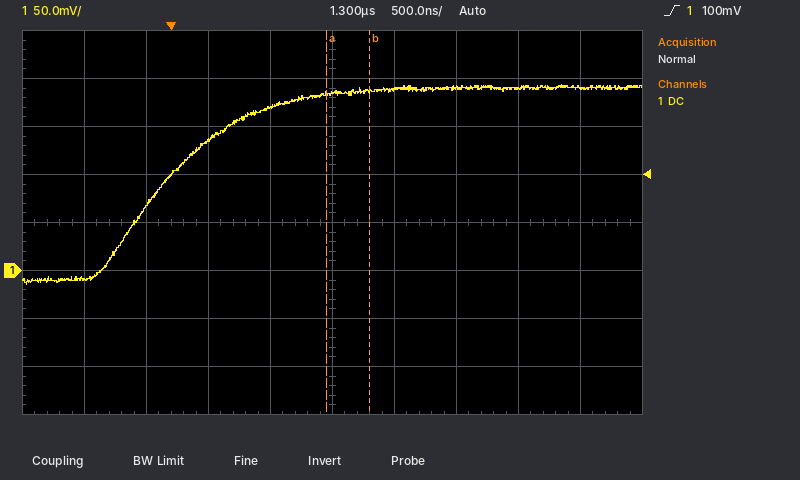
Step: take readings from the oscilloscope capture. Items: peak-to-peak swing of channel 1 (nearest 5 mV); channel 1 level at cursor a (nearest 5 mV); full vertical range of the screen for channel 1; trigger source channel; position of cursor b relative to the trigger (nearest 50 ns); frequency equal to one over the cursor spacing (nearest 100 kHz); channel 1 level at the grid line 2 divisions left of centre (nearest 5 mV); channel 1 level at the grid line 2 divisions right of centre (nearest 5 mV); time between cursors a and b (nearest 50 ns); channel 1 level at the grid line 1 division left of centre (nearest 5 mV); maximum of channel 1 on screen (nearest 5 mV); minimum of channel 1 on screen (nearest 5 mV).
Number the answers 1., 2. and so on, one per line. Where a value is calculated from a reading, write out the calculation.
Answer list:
1. 195 mV − (-15 mV) = 210 mV
2. 185 mV
3. 400 mV
4. channel 1
5. +1.60 µs
6. 1 / 350 ns ≈ 2.9 MHz
7. 135 mV
8. 190 mV
9. 350 ns
10. 170 mV
11. 195 mV
12. -15 mV
